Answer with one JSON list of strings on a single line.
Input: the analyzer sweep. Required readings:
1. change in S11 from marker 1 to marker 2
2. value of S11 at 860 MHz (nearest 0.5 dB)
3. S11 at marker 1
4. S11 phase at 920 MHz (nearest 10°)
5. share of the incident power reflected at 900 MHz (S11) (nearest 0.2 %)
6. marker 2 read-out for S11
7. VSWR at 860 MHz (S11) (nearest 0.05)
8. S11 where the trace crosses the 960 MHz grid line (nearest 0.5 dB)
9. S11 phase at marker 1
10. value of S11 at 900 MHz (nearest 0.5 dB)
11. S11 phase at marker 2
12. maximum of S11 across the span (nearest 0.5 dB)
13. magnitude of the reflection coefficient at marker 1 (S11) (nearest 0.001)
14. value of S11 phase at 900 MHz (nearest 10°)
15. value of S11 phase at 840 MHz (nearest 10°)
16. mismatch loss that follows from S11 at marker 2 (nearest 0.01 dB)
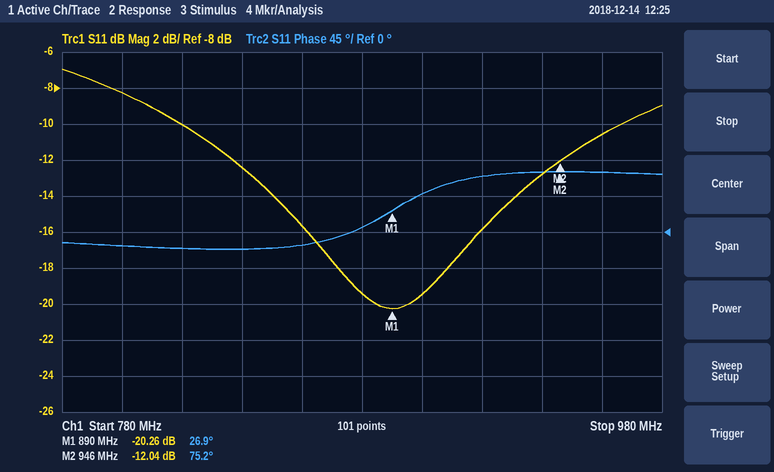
["8.22 dB", "-15.5 dB", "-20.26 dB", "70°", "1.2 %", "-12.04 dB", "1.40", "-10.5 dB", "26.9°", "-19.5 dB", "75.2°", "-7.0 dB", "0.097", "50°", "-20°", "0.28 dB"]
